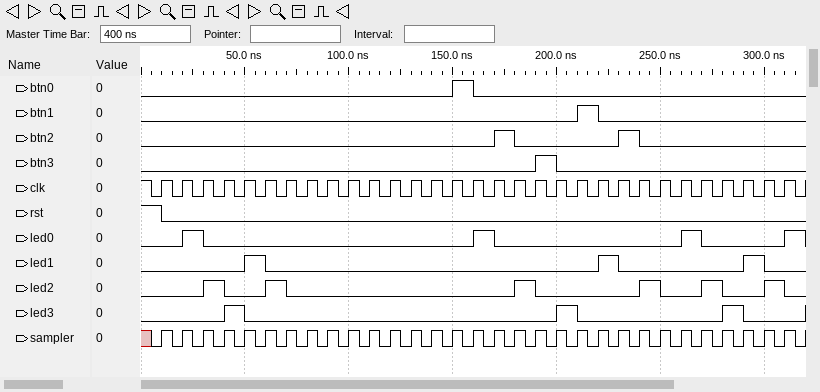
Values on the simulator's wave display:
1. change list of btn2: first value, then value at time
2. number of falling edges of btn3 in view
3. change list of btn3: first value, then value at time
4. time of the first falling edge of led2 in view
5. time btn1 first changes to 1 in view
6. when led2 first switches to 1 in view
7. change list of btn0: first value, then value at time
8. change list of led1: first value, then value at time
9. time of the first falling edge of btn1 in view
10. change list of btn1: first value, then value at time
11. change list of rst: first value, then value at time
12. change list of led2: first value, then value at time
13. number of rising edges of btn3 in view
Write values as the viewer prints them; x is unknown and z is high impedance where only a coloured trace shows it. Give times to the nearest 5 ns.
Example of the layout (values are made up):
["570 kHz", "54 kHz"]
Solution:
["0, 1 at 170 ns, 0 at 180 ns, 1 at 230 ns, 0 at 240 ns", "1", "0, 1 at 190 ns, 0 at 200 ns", "40 ns", "210 ns", "30 ns", "0, 1 at 150 ns, 0 at 160 ns", "0, 1 at 50 ns, 0 at 60 ns, 1 at 220 ns, 0 at 230 ns, 1 at 290 ns, 0 at 300 ns", "220 ns", "0, 1 at 210 ns, 0 at 220 ns", "1, 0 at 10 ns", "0, 1 at 30 ns, 0 at 40 ns, 1 at 60 ns, 0 at 70 ns, 1 at 180 ns, 0 at 190 ns, 1 at 240 ns, 0 at 250 ns, 1 at 270 ns, 0 at 280 ns, 1 at 300 ns, 0 at 310 ns", "1"]
